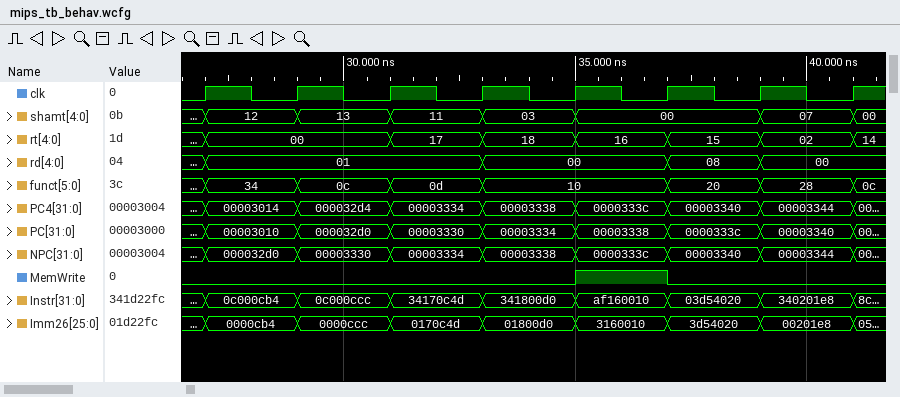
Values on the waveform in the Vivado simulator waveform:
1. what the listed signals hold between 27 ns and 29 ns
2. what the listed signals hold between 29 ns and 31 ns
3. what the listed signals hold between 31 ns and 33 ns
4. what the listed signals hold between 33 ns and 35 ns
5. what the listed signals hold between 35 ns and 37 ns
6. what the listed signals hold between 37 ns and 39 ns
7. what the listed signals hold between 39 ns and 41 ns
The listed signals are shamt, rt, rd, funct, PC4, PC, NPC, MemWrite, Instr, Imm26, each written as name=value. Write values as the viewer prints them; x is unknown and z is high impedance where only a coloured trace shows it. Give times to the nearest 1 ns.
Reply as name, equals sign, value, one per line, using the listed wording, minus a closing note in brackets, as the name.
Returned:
what the listed signals hold between 27 ns and 29 ns = shamt=12, rt=00, rd=01, funct=34, PC4=00003014, PC=00003010, NPC=000032d0, MemWrite=0, Instr=0c000cb4, Imm26=0000cb4
what the listed signals hold between 29 ns and 31 ns = shamt=13, rt=00, rd=01, funct=0c, PC4=000032d4, PC=000032d0, NPC=00003330, MemWrite=0, Instr=0c000ccc, Imm26=0000ccc
what the listed signals hold between 31 ns and 33 ns = shamt=11, rt=17, rd=01, funct=0d, PC4=00003334, PC=00003330, NPC=00003334, MemWrite=0, Instr=34170c4d, Imm26=0170c4d
what the listed signals hold between 33 ns and 35 ns = shamt=03, rt=18, rd=00, funct=10, PC4=00003338, PC=00003334, NPC=00003338, MemWrite=0, Instr=341800d0, Imm26=01800d0
what the listed signals hold between 35 ns and 37 ns = shamt=00, rt=16, rd=00, funct=10, PC4=0000333c, PC=00003338, NPC=0000333c, MemWrite=1, Instr=af160010, Imm26=3160010
what the listed signals hold between 37 ns and 39 ns = shamt=00, rt=15, rd=08, funct=20, PC4=00003340, PC=0000333c, NPC=00003340, MemWrite=0, Instr=03d54020, Imm26=3d54020
what the listed signals hold between 39 ns and 41 ns = shamt=07, rt=02, rd=00, funct=28, PC4=00003344, PC=00003340, NPC=00003344, MemWrite=0, Instr=340201e8, Imm26=00201e8
